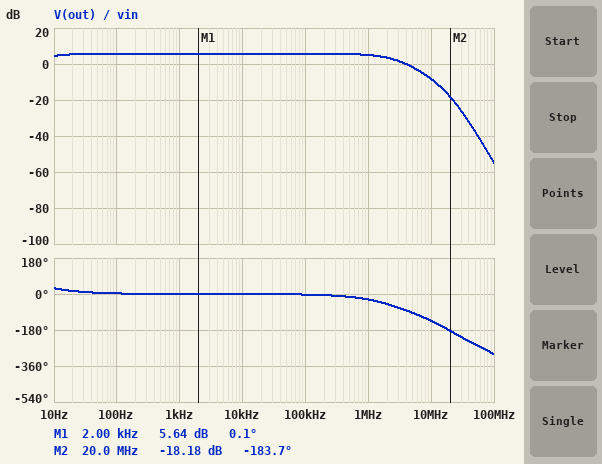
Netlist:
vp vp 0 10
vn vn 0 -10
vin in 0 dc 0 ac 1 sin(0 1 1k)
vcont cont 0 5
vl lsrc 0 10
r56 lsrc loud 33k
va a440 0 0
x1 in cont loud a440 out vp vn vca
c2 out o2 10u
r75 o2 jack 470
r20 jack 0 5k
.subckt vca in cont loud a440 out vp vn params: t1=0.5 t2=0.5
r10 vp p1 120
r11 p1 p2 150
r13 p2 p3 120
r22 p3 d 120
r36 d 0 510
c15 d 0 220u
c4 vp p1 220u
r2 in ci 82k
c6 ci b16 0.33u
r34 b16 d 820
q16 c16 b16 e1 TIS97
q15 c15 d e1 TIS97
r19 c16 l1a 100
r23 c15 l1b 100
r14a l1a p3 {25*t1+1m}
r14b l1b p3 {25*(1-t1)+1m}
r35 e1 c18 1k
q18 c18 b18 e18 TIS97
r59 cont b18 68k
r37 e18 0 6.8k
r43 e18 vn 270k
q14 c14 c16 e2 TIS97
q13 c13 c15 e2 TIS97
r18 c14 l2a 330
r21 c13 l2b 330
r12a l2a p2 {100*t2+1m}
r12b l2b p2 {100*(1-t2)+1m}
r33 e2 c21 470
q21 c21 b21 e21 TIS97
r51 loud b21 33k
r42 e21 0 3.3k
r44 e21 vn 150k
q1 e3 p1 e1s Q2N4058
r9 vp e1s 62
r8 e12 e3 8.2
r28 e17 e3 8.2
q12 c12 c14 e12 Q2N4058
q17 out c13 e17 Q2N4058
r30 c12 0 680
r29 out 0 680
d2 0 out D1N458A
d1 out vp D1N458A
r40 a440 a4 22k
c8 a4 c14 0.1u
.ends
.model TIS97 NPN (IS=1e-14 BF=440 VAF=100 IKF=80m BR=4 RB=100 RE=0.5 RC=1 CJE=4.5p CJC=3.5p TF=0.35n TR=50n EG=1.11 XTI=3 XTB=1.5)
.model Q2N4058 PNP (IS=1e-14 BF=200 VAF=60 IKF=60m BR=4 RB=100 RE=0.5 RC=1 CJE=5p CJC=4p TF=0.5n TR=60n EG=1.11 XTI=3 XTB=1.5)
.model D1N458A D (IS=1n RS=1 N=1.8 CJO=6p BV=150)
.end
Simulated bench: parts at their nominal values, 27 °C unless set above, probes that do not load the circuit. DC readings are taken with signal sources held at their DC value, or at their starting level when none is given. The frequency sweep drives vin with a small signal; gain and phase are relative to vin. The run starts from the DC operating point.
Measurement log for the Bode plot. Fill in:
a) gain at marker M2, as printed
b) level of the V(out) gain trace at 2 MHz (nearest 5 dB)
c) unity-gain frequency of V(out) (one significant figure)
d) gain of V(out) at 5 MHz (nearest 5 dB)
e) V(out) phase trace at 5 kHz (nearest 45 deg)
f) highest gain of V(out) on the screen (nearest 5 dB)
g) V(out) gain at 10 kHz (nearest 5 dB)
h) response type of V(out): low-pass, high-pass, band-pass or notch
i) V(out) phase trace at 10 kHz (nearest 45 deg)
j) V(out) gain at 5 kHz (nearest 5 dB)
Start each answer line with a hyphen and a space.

- -18.18 dB
- 5 dB
- 4 MHz
- 0 dB
- 0 deg
- 5 dB
- 5 dB
- low-pass
- 0 deg
- 5 dB
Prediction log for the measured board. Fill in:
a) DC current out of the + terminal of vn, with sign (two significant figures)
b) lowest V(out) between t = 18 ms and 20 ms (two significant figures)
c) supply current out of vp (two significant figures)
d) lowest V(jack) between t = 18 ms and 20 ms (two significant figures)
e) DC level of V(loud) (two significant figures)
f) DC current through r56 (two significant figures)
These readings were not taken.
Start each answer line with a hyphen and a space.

- -150 µA
- 1.4 V
- 21 mA
- -1.6 V
- 7.6 V
- 74 µA
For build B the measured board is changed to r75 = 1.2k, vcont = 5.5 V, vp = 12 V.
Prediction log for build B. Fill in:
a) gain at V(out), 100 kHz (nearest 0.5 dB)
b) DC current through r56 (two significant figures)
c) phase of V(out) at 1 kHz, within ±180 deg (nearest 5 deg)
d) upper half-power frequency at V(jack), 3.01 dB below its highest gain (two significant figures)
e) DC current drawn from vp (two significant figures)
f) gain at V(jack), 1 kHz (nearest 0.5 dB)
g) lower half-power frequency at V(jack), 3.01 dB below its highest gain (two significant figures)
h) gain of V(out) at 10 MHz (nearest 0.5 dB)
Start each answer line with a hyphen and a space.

- 10.0 dB
- 59 µA
- 0 deg
- 2.3 MHz
- 27 mA
- 8.0 dB
- 6.5 Hz
- -5.0 dB
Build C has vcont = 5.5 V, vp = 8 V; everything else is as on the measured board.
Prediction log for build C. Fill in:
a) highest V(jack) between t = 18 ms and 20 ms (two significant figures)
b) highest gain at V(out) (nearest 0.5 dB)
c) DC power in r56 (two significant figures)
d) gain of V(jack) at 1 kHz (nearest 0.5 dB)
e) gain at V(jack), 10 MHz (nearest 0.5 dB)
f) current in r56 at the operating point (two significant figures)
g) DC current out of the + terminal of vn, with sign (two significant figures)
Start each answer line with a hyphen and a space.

- 800 mV
- -0.5 dB
- 260 µW
- -1.5 dB
- -14.0 dB
- 89 µA
- -140 µA
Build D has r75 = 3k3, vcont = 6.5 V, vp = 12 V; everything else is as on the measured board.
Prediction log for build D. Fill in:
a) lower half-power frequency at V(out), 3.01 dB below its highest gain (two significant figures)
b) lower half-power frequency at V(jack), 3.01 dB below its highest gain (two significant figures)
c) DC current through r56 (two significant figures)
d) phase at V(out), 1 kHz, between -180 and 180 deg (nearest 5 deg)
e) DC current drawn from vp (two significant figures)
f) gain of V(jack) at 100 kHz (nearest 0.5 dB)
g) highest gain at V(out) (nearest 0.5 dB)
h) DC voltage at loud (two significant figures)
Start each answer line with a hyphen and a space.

- 5.7 Hz
- 6.2 Hz
- 59 µA
- 0 deg
- 27 mA
- 5.5 dB
- 10.0 dB
- 8.1 V
